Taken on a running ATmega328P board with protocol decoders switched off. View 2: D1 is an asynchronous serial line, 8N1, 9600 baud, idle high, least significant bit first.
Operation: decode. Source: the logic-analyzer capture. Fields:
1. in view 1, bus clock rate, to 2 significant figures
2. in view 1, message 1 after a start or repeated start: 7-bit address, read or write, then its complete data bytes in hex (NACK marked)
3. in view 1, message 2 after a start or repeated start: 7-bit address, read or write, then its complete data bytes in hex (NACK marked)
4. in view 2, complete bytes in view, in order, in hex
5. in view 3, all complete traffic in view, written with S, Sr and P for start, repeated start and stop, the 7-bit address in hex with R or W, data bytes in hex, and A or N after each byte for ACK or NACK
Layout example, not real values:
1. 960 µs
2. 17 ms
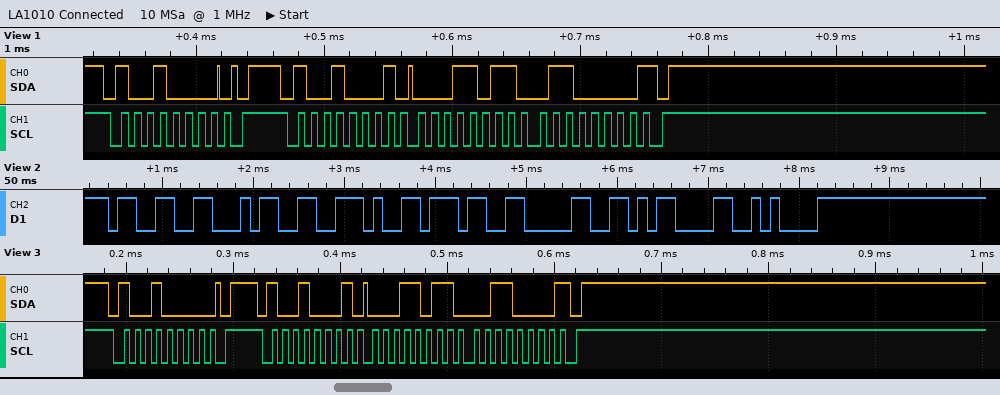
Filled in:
1. 100 kHz
2. 0x48 write
3. 0x48 read: 1B 60 NACK
4. 33 34 2E 37 30 0D 0A
5. S 48W A P S 48R A 1B A 30 N P
